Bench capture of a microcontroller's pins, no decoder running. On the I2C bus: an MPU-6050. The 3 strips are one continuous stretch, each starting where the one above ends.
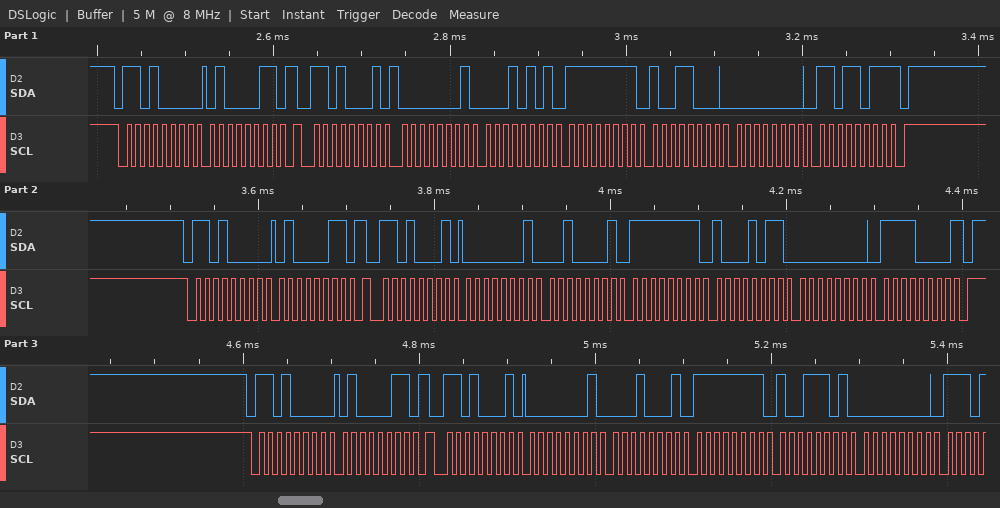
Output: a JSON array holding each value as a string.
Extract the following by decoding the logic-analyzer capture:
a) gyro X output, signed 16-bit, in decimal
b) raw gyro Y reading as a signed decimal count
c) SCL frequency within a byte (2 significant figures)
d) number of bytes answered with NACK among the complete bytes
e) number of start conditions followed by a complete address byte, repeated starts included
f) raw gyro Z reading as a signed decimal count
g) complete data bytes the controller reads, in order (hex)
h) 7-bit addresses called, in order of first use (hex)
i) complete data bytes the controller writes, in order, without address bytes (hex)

["277", "-104", "100 kHz", "2", "6", "219", "01 15 FF 98 00 DB 01 21 FF 8B 00 F0 01 11 FF 9D 00", "0x68", "43 43 43"]
